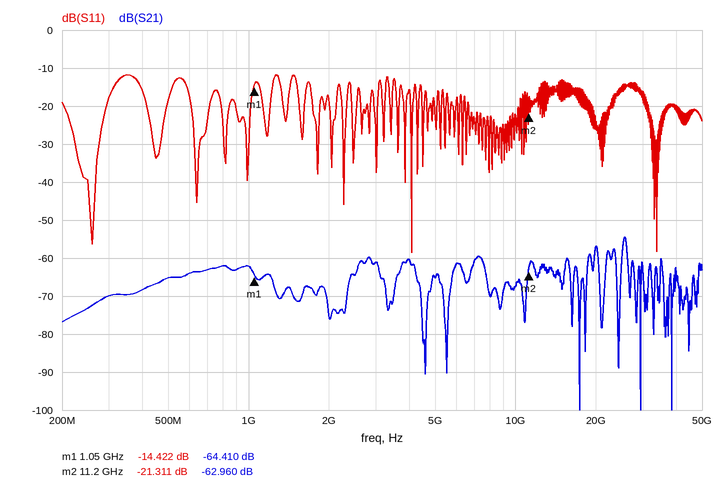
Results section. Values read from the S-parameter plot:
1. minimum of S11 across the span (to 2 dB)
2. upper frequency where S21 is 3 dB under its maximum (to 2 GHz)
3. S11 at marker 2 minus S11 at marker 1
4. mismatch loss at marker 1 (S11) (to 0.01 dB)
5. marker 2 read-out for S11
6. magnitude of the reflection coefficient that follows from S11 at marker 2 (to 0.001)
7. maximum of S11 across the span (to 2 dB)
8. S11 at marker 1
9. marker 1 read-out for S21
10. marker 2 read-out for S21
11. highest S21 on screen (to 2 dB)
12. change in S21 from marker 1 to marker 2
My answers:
-58 dB
26 GHz
-6.889 dB
0.16 dB
-21.311 dB
0.086
-12 dB
-14.422 dB
-64.410 dB
-62.960 dB
-54 dB
1.450 dB
